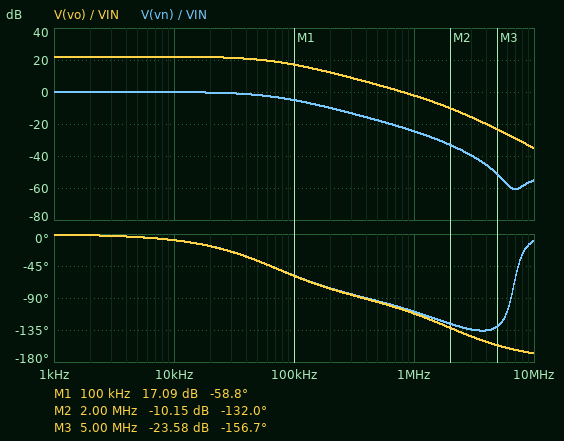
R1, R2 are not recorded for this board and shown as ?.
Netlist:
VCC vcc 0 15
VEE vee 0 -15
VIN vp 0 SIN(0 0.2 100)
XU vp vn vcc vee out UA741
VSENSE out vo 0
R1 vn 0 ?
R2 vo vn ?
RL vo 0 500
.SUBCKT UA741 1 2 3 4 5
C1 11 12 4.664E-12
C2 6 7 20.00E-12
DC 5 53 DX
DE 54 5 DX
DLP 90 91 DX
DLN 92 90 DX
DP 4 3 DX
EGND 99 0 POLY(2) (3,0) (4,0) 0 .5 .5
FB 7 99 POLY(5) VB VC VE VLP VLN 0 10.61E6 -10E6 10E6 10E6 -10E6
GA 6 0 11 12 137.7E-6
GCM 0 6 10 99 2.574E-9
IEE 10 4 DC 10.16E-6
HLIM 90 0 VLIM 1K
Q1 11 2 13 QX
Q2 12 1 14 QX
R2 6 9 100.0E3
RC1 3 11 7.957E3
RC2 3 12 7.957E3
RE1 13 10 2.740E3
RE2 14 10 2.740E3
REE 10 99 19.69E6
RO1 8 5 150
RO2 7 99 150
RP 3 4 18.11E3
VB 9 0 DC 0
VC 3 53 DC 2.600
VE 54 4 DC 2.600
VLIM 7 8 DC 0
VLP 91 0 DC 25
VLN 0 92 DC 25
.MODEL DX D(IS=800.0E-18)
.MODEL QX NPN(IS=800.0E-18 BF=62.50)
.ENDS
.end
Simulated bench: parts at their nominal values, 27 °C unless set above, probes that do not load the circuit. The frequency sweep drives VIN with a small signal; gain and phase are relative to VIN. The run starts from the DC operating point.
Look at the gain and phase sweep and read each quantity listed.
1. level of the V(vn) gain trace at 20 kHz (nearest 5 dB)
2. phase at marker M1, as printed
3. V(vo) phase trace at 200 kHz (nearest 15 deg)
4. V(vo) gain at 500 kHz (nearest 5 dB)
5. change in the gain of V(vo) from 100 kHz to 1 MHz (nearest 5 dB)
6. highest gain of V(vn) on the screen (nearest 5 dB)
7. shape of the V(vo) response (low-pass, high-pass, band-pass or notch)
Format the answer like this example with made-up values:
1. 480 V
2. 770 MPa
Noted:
1. 0 dB
2. -58.8 deg
3. -75 deg
4. 5 dB
5. -20 dB
6. 0 dB
7. low-pass
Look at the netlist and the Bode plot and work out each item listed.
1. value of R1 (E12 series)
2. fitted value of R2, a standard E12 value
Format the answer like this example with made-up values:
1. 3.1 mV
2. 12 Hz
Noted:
1. 3.3 kΩ
2. 39 kΩ
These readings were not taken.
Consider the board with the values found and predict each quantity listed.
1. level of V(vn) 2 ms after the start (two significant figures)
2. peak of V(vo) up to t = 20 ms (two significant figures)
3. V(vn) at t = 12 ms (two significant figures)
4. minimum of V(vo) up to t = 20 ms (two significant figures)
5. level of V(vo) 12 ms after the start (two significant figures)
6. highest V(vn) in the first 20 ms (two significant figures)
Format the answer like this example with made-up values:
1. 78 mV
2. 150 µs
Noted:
1. 190 mV
2. 2.6 V
3. 190 mV
4. -2.6 V
5. 2.4 V
6. 200 mV
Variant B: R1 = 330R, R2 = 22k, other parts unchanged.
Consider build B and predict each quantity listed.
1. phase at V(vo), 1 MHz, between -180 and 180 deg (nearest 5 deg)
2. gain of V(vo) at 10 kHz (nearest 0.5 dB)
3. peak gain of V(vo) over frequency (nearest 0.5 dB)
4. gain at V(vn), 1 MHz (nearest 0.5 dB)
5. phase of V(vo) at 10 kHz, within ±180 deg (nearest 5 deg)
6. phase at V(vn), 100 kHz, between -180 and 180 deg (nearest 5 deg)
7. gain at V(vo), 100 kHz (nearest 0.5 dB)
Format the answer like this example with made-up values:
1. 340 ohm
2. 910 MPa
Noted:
1. -115 deg
2. 34.5 dB
3. 36.5 dB
4. -39.0 dB
5. -40 deg
6. -85 deg
7. 18.5 dB
